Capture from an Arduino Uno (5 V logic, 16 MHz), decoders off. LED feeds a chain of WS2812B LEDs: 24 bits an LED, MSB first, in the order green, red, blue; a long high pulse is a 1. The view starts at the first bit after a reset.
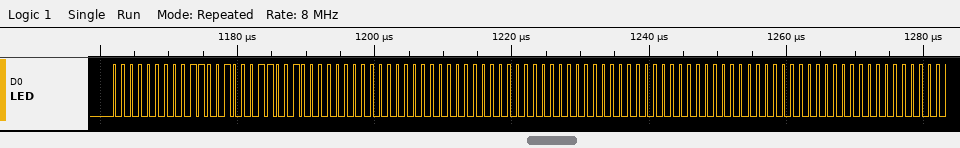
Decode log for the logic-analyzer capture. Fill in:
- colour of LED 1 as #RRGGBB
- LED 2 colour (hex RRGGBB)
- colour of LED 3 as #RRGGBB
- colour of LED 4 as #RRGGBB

#640064
#000000
#000000
#000000
